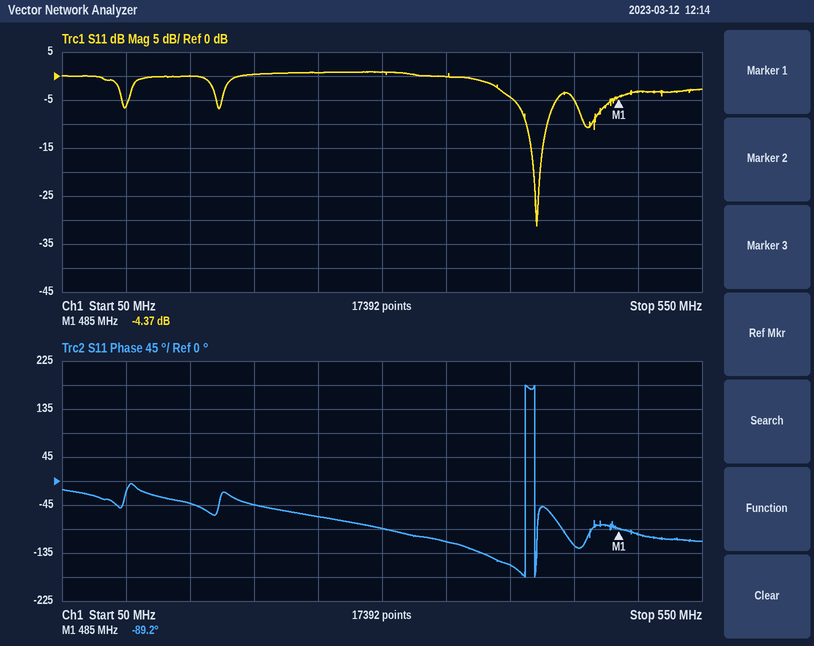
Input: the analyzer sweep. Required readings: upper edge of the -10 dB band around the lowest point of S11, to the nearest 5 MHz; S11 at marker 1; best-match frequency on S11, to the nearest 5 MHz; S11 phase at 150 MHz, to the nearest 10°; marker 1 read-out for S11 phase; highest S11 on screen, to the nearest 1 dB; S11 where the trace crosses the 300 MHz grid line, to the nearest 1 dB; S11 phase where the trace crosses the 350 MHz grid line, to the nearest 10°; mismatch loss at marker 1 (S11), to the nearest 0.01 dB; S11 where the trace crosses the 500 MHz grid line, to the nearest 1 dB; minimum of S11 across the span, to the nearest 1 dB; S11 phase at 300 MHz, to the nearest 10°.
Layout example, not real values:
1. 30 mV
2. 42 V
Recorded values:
1. 430 MHz
2. -4.37 dB
3. 420 MHz
4. -40°
5. -89.2°
6. 1 dB
7. 1 dB
8. -110°
9. 1.98 dB
10. -3 dB
11. -31 dB
12. -90°
